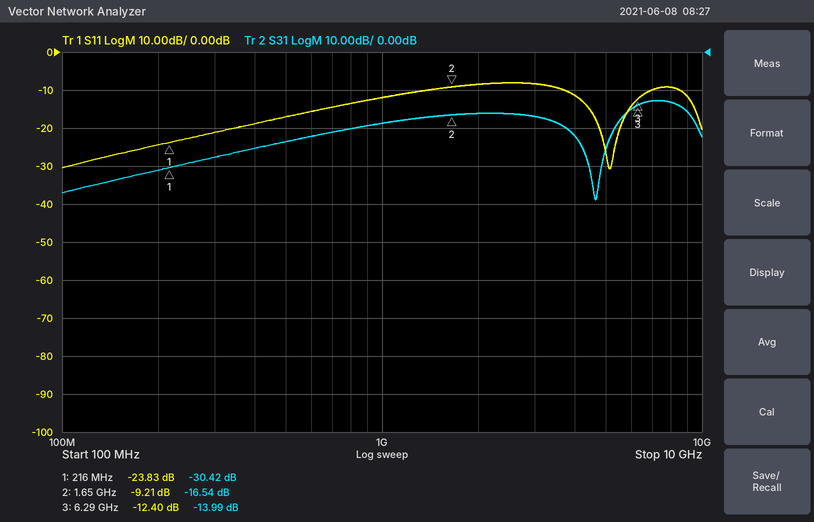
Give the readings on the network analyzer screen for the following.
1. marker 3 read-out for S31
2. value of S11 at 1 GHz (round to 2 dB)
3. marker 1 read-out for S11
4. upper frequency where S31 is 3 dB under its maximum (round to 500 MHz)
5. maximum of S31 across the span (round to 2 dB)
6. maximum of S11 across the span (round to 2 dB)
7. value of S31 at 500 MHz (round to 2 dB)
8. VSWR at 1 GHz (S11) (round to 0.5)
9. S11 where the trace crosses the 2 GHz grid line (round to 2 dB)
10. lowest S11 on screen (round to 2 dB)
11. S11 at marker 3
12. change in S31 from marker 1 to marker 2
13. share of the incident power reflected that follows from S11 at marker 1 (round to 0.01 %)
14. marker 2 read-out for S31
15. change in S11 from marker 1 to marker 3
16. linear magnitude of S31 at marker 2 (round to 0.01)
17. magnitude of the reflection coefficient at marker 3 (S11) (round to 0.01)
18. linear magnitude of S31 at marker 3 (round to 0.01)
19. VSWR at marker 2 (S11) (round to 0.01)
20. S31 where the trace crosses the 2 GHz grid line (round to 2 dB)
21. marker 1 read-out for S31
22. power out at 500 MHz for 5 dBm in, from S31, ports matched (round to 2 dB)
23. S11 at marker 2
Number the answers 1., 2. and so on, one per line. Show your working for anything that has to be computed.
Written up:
1. -13.99 dB
2. -12 dB
3. -23.83 dB
4. 9.0 GHz
5. -12 dB
6. -8 dB
7. -24 dB
8. |Γ| = 10^(-12/20) = 0.2512; VSWR = (1 + 0.2512)/(1 − 0.2512) ≈ 1.67, so 1.5 to the nearest 0.5
9. -8 dB
10. -30 dB
11. -12.40 dB
12. -16.54 − (-30.42) = 13.88 dB
13. 10^(-23.83/10) ≈ 0.41 %
14. -16.54 dB
15. -12.4 − (-23.83) = 11.43 dB
16. 10^(-16.54/20) ≈ 0.15
17. 10^(-12.4/20) ≈ 0.24
18. 10^(-13.99/20) ≈ 0.20
19. (1 + 0.3463)/(1 − 0.3463) ≈ 2.06
20. -16 dB
21. -30.42 dB
22. 5 dBm + (-24 dB) = -18 dBm
23. -9.21 dB
